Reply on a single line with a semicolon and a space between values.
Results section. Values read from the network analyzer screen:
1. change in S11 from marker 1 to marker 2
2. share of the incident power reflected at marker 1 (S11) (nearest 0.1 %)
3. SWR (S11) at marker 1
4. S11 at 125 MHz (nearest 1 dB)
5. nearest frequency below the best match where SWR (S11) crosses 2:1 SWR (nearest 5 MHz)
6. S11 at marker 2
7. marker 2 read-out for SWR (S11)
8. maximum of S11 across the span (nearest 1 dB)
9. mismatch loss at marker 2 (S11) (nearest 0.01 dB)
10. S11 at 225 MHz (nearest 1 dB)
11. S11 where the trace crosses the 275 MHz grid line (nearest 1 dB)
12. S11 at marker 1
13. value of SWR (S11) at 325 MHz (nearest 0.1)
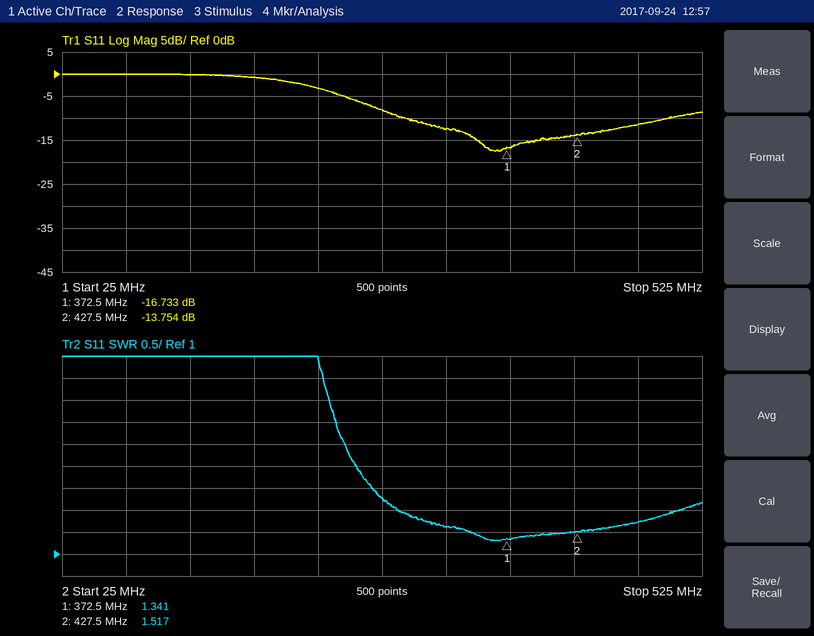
2.979 dB; 2.1 %; 1.341; 0 dB; 285 MHz; -13.754 dB; 1.517; 0 dB; 0.19 dB; -3 dB; -8 dB; -16.733 dB; 1.6
